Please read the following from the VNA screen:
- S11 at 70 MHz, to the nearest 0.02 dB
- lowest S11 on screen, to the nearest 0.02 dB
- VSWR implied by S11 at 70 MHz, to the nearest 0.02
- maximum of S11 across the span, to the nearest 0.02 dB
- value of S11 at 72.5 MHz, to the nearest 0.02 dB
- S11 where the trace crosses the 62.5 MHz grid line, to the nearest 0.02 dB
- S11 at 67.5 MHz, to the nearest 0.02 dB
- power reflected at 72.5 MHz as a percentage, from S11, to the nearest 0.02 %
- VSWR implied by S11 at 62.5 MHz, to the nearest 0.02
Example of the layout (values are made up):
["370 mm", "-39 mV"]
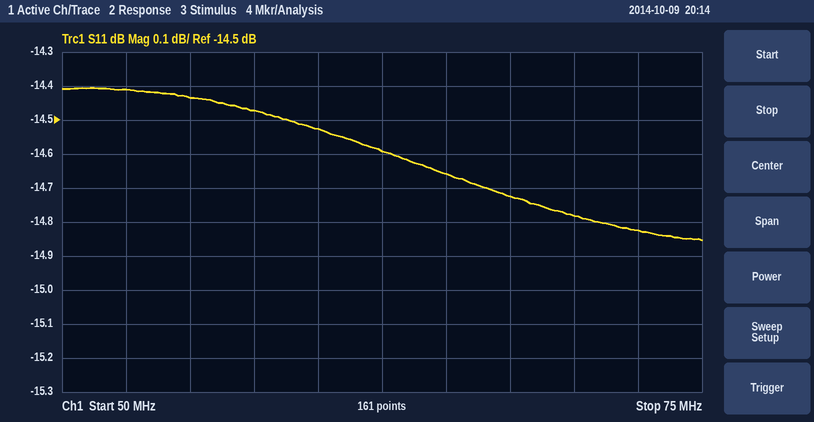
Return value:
["-14.78 dB", "-14.86 dB", "1.44", "-14.40 dB", "-14.82 dB", "-14.60 dB", "-14.72 dB", "3.30 %", "1.46"]
